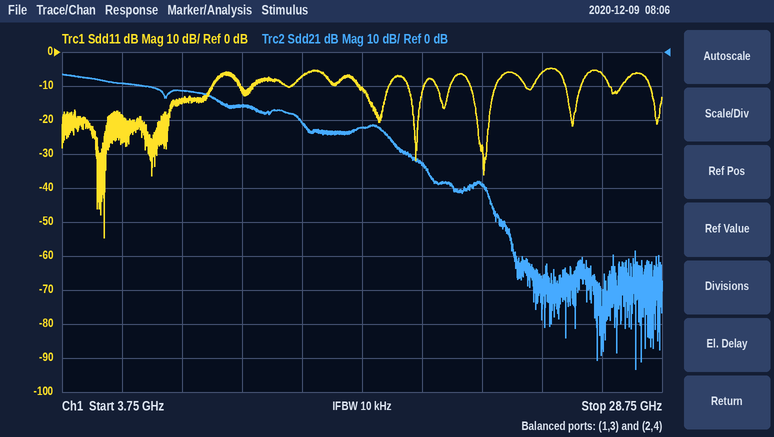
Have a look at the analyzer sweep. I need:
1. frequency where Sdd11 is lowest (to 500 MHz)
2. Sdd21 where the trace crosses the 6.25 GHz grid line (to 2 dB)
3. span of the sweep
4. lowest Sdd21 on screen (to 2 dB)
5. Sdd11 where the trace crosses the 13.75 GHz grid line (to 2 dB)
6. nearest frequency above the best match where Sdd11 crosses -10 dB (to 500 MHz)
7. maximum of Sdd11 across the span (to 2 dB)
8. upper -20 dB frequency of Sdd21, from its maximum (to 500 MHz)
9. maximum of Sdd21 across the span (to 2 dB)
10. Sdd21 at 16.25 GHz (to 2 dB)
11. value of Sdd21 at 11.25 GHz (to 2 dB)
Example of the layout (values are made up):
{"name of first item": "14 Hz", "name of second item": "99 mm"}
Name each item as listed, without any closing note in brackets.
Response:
{"frequency where Sdd11 is lowest": "5.5 GHz", "Sdd21 where the trace crosses the 6.25 GHz grid line": "-10 dB", "span of the sweep": "25 GHz", "lowest Sdd21 on screen": "-94 dB", "Sdd11 where the trace crosses the 13.75 GHz grid line": "-8 dB", "nearest frequency above the best match where Sdd11 crosses -10 dB": "10.0 GHz", "maximum of Sdd11 across the span": "-4 dB", "upper -20 dB frequency of Sdd21, from its maximum": "17.5 GHz", "maximum of Sdd21 across the span": "-6 dB", "Sdd21 at 16.25 GHz": "-22 dB", "value of Sdd21 at 11.25 GHz": "-16 dB"}
